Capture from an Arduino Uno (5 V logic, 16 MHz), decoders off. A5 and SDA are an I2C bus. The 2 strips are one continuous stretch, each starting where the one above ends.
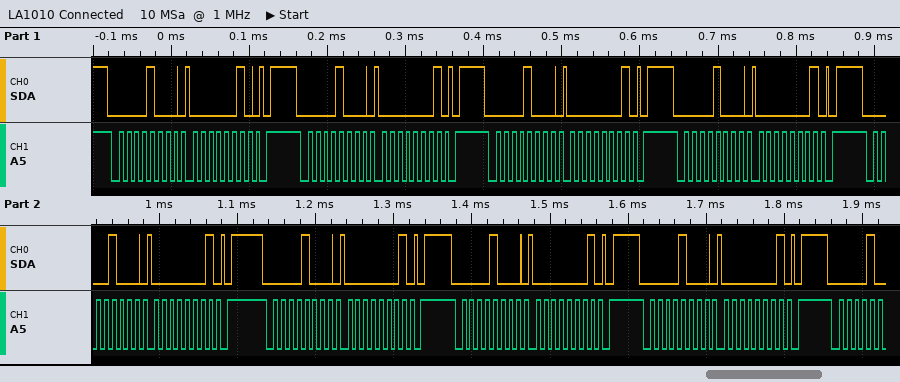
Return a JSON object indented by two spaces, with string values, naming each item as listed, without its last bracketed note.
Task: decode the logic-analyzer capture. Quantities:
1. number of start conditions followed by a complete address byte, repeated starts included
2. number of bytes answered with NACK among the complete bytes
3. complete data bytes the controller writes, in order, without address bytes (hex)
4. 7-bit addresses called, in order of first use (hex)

{
  "number of start conditions followed by a complete address byte, repeated starts included": "8",
  "number of bytes answered with NACK among the complete bytes": "0",
  "complete data bytes the controller writes, in order, without address bytes": "02 01 01 01 01 01 01 01",
  "7-bit addresses called, in order of first use": "0x04"
}
